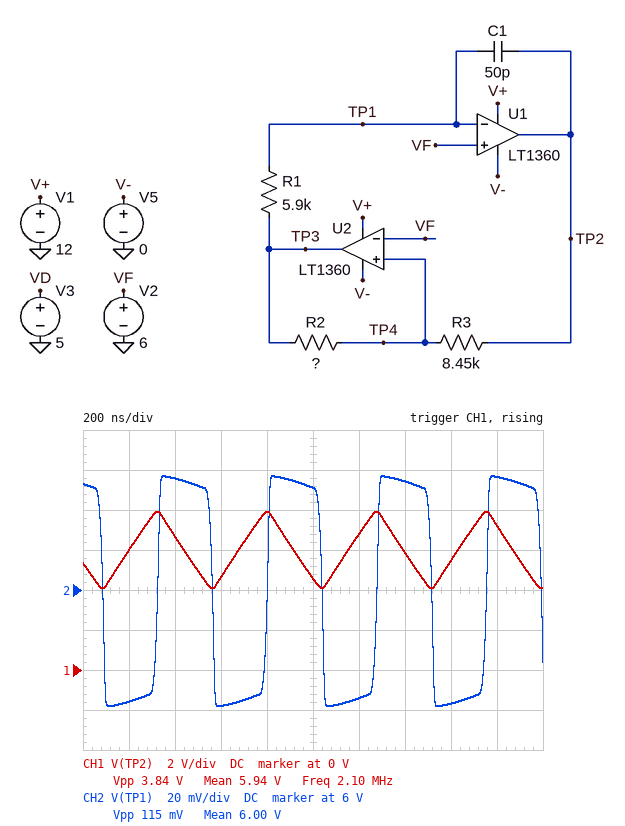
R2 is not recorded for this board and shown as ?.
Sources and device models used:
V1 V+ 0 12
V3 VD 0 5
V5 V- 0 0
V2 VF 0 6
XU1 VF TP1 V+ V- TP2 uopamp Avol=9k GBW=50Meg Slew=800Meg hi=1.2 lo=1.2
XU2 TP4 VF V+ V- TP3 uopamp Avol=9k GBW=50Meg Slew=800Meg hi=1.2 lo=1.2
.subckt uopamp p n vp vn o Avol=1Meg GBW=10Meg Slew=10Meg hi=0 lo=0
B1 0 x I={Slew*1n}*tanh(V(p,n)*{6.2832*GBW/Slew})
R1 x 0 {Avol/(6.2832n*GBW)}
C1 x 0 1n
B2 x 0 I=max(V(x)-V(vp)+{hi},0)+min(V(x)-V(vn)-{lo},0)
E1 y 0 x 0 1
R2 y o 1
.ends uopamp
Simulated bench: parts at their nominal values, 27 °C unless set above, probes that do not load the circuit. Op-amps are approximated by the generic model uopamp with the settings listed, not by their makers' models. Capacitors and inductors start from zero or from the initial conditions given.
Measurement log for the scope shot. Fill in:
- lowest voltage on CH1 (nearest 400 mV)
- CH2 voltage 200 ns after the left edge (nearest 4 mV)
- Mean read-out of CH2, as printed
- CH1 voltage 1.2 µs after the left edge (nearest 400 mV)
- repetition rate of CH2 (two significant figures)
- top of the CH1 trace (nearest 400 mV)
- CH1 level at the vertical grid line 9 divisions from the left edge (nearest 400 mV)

4.0 V
5.944 V
6.00 V
6.8 V
2.1 MHz
8.0 V
7.2 V
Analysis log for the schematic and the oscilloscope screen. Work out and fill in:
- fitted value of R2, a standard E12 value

27 kΩ
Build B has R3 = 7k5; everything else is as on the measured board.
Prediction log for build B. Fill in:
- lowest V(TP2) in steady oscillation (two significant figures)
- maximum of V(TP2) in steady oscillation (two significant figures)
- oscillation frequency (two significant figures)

4.2 V
7.8 V
2.3 MHz
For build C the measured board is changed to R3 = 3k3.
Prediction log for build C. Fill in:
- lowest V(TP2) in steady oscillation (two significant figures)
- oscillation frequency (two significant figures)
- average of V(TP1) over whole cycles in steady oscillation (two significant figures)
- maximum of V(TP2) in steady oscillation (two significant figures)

4.9 V
3.4 MHz
6.0 V
7.1 V
